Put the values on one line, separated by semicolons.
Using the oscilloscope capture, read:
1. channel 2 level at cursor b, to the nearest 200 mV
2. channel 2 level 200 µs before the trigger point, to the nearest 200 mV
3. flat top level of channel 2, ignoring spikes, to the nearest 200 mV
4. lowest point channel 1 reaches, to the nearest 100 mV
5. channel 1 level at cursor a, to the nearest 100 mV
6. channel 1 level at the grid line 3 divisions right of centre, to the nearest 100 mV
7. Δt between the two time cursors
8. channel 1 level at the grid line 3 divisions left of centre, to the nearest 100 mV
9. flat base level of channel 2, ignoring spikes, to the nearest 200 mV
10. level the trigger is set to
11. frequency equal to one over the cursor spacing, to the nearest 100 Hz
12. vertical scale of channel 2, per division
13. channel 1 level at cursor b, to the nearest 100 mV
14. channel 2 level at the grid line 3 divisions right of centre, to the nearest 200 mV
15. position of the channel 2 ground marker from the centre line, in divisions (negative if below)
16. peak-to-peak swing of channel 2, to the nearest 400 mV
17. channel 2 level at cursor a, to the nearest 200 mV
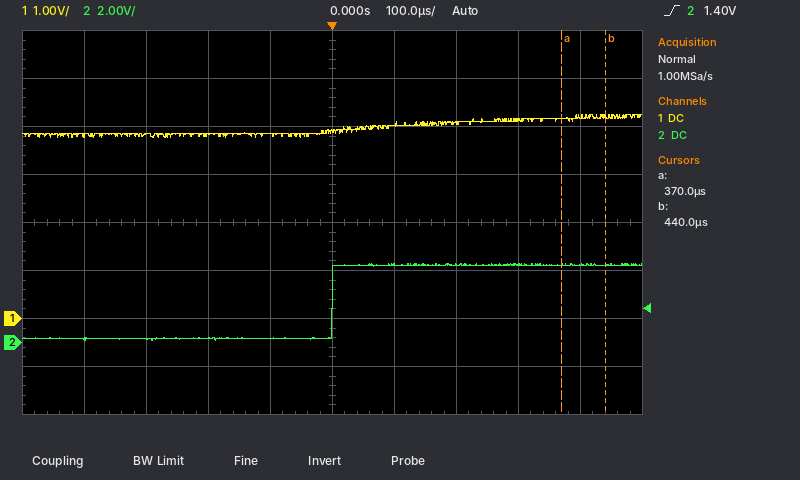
3.2 V; 200 mV; 3.2 V; 3.8 V; 4.2 V; 4.1 V; 70 µs; 3.8 V; 200 mV; 1.40 V; 14.3 kHz; 2 V; 4.2 V; 3.2 V; -2.5 div; 3.2 V; 3.2 V
